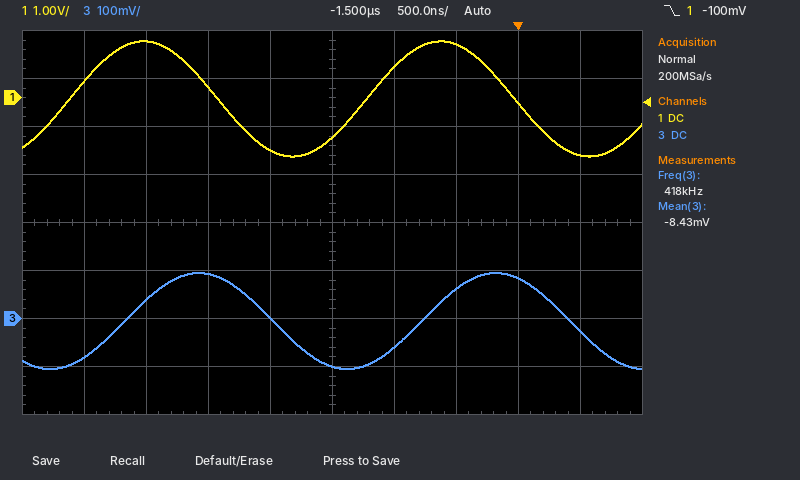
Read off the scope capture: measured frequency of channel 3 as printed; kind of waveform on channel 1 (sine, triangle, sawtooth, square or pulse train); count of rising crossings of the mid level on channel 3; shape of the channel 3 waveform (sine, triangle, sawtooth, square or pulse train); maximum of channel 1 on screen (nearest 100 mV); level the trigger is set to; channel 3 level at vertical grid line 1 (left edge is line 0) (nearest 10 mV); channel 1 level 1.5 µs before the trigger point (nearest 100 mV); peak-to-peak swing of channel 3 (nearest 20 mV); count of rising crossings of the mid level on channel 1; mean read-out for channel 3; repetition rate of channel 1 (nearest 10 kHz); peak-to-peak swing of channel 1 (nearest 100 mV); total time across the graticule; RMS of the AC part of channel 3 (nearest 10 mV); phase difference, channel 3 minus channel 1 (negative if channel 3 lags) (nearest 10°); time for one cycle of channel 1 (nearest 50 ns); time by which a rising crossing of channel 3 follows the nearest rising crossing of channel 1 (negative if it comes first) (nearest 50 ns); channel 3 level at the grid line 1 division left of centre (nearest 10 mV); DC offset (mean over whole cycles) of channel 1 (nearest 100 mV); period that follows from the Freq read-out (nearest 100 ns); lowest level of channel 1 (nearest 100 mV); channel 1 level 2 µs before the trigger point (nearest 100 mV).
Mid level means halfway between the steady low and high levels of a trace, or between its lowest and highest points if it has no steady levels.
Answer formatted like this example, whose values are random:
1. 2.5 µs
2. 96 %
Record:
1. 418 kHz
2. sine
3. 2
4. sine
5. 1.2 V
6. -100 mV
7. -80 mV
8. -800 mV
9. 200 mV
10. 2
11. -8.43 mV
12. 420 kHz
13. 2.4 V
14. 5 µs
15. 70 mV
16. -70°
17. 2.40 µs
18. +450 ns
19. 0 mV
20. 0.0 V
21. 2.4 µs
22. -1.2 V
23. -1.1 V
